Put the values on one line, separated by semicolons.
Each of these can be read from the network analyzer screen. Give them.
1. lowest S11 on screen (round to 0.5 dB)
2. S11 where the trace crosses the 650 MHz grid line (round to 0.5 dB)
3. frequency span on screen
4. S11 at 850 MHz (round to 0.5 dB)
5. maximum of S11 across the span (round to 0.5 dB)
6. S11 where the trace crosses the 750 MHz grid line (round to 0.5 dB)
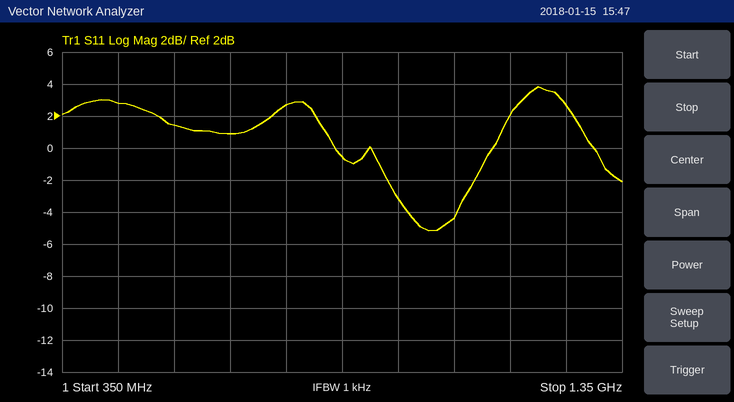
-5.0 dB; 1.0 dB; 1 GHz; -0.5 dB; 4.0 dB; 2.5 dB
